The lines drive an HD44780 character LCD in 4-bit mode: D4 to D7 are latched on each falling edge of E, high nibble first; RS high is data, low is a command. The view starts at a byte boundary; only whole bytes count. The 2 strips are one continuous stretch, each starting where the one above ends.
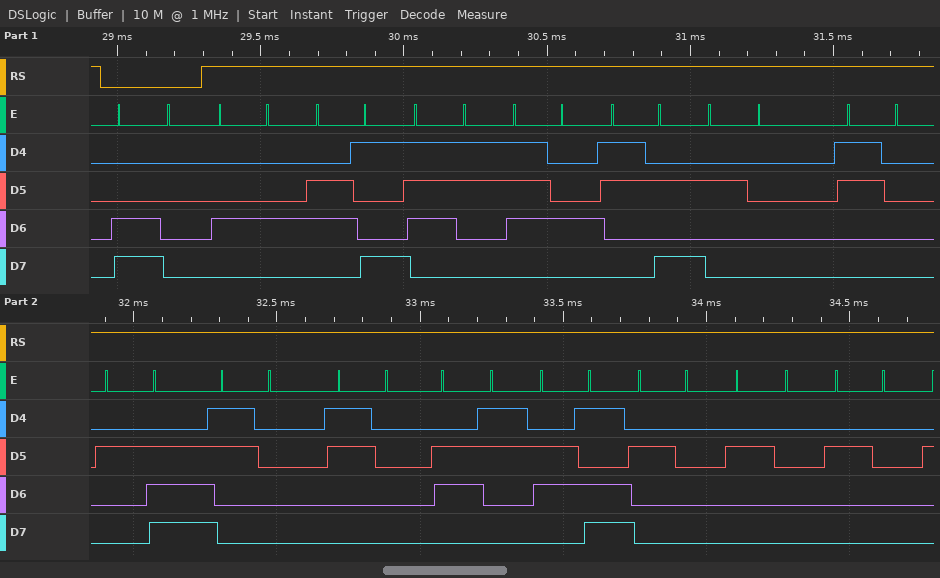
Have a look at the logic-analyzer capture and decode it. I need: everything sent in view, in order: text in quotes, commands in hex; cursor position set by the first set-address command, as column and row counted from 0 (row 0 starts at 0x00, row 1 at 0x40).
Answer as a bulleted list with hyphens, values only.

- 0xC0 "Dist: 0.00cm   "
- column 0, row 1
